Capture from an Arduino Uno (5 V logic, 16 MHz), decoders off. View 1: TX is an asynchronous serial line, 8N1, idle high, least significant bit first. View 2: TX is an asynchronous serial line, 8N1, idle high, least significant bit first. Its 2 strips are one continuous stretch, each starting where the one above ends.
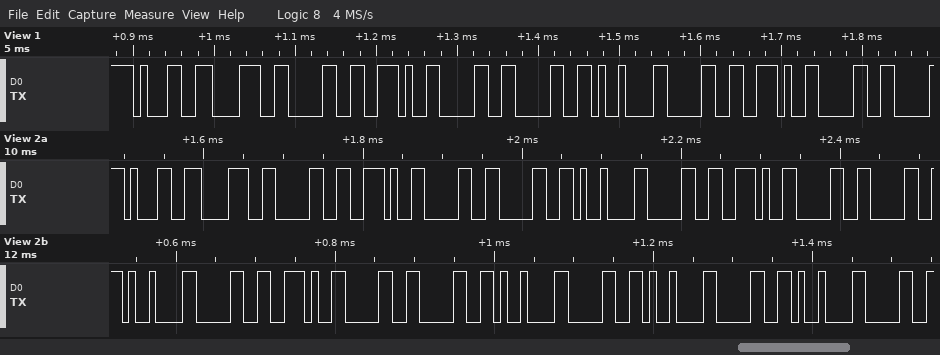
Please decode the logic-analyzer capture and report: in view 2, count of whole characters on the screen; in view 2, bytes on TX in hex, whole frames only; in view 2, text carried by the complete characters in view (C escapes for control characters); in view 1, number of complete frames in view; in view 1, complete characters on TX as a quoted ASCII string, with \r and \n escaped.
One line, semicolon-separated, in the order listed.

22; 31 38 30 2E 30 30 09 30 2E 30 30 09 30 2E 30 30 09 30 09 30 09 30; "180.00\t0.00\t0.00\t0\t0\t0"; 10; "180.00\t0.0"
